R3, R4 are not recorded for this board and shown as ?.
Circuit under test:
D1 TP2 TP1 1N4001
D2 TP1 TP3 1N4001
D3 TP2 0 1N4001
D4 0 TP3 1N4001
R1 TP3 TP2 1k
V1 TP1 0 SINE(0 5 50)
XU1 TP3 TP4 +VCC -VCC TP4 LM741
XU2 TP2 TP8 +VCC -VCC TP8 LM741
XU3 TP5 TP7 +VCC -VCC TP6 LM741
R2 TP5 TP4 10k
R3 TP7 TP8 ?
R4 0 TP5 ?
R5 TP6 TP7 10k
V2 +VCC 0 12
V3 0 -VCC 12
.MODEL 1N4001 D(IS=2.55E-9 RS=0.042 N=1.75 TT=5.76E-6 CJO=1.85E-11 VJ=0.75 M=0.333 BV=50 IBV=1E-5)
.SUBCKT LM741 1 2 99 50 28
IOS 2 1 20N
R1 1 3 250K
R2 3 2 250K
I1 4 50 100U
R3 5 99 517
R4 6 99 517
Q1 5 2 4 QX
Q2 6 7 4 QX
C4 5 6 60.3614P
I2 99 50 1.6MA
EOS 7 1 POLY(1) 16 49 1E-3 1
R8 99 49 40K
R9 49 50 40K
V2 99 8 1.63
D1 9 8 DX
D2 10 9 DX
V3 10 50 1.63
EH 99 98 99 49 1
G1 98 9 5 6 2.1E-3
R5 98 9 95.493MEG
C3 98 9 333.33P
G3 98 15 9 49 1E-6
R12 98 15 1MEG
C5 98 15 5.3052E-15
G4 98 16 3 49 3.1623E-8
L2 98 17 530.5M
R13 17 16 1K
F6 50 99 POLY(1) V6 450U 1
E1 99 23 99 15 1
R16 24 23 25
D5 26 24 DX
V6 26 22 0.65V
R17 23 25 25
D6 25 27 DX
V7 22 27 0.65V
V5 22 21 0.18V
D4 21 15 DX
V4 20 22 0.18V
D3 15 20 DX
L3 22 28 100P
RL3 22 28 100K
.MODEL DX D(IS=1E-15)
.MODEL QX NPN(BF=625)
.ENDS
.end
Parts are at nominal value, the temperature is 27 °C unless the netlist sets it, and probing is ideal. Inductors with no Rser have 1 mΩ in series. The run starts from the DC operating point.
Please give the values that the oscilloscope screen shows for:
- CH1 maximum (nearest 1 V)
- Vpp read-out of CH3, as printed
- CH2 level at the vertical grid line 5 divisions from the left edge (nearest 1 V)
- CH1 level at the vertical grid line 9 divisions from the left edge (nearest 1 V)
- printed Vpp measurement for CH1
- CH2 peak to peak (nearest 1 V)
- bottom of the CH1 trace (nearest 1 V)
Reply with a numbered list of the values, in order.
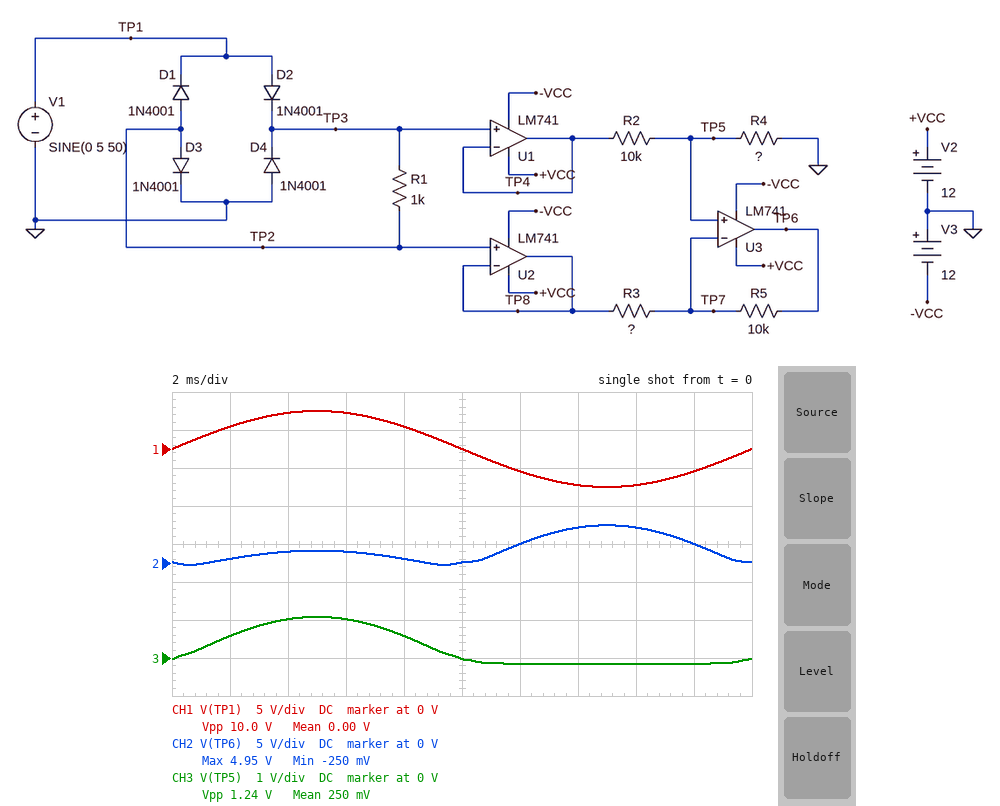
1. 5 V
2. 1.24 V
3. 0 V
4. -3 V
5. 10.0 V
6. 5 V
7. -5 V
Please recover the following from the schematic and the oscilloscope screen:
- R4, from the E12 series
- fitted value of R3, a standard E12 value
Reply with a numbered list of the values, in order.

1. 3.3 kΩ
2. 8.2 kΩ
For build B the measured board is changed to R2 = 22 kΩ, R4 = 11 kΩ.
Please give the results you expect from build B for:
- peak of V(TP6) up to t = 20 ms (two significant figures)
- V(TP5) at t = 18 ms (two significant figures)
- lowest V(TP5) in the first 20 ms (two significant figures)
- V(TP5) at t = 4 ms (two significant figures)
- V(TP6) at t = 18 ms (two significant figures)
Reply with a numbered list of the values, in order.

1. 4.8 V
2. -200 mV
3. -210 mV
4. 1.4 V
5. 2.4 V
